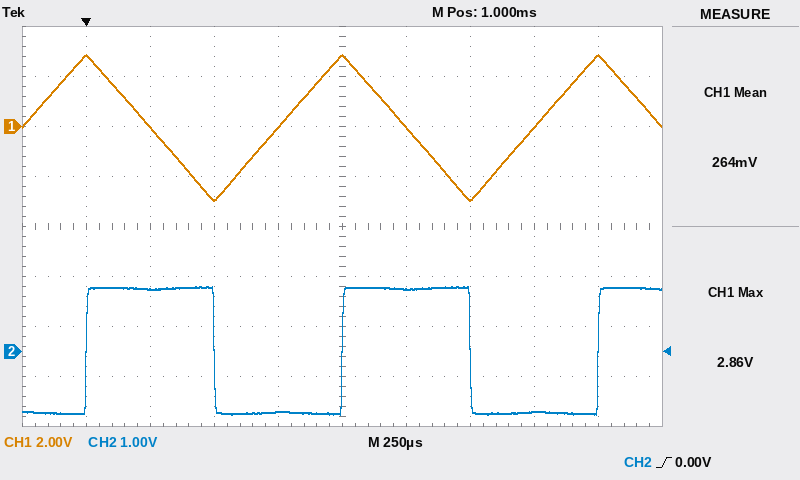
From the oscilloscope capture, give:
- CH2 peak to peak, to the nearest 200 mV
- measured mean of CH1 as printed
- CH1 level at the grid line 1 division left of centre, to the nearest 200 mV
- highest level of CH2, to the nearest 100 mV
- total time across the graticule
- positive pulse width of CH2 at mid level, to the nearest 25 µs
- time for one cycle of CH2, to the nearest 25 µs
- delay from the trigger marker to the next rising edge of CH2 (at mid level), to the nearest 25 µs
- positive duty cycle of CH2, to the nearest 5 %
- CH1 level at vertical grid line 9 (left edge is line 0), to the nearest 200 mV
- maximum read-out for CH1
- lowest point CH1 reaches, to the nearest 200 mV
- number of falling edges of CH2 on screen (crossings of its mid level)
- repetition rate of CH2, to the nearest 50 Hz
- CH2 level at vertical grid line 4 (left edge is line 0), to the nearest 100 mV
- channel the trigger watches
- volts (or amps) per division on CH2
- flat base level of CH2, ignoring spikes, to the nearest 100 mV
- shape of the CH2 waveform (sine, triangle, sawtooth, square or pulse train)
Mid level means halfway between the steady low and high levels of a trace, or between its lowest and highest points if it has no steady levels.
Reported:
2.6 V
264 mV
0.0 V
1.3 V
2.5 ms
500 µs
1.000 ms
1.000 ms
50 %
2.8 V
2.86 V
-3.0 V
2
1.00 kHz
-1.2 V
CH2
1 V
-1.2 V
square
